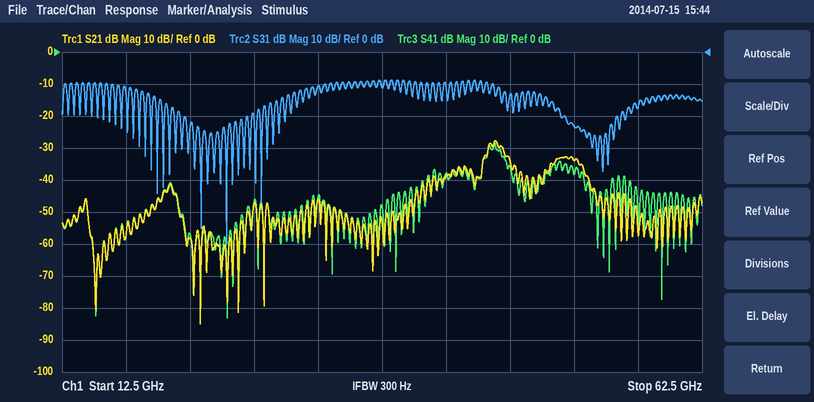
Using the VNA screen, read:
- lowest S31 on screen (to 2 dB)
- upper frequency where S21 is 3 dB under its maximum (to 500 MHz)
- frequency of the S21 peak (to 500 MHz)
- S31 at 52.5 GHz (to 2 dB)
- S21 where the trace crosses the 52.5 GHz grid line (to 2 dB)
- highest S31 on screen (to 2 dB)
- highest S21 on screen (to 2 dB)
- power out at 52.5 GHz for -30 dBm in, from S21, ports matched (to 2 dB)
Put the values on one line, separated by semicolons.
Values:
-60 dB; 47.0 GHz; 46.5 GHz; -24 dB; -34 dB; -8 dB; -28 dB; -64 dBm
